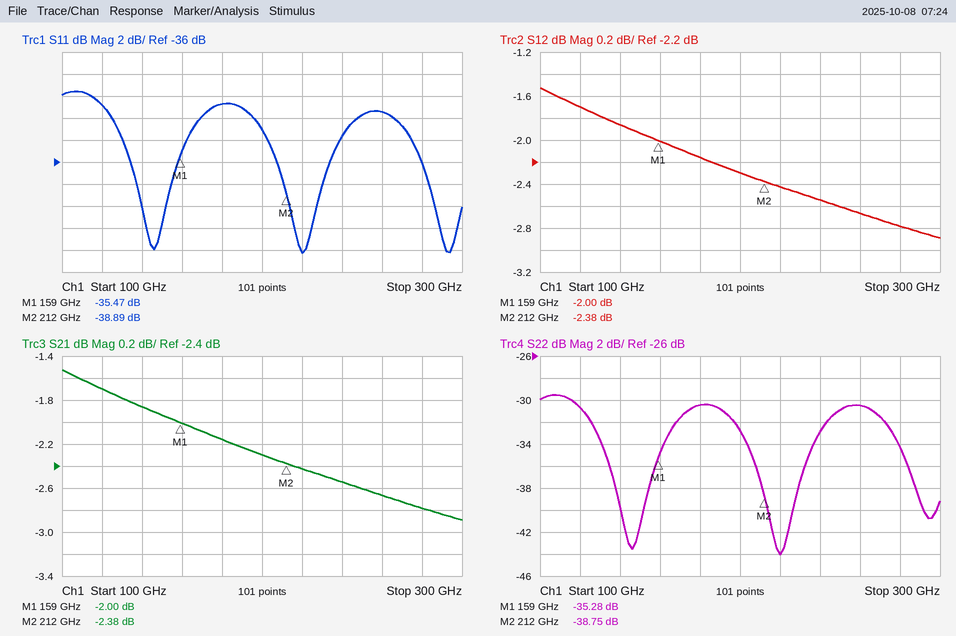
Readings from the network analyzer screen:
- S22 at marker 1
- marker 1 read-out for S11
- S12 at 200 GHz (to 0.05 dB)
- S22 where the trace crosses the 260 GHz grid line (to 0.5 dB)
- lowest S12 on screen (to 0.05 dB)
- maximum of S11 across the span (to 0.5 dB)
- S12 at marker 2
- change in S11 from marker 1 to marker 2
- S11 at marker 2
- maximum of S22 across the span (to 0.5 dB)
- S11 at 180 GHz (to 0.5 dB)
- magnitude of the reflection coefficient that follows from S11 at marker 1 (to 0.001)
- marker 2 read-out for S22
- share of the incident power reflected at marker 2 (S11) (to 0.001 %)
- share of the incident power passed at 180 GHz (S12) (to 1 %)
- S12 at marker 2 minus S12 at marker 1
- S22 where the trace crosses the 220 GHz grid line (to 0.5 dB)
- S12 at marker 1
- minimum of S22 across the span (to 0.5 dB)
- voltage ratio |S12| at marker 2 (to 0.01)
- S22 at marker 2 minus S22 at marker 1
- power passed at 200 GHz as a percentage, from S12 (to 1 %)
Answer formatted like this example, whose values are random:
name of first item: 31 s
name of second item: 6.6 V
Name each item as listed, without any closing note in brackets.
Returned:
S22 at marker 1: -35.28 dB
marker 1 read-out for S11: -35.47 dB
S12 at 200 GHz: -2.30 dB
S22 where the trace crosses the 260 GHz grid line: -30.5 dB
lowest S12 on screen: -2.90 dB
maximum of S11 across the span: -29.5 dB
S12 at marker 2: -2.38 dB
change in S11 from marker 1 to marker 2: -3.42 dB
S11 at marker 2: -38.89 dB
maximum of S22 across the span: -29.5 dB
S11 at 180 GHz: -30.5 dB
magnitude of the reflection coefficient that follows from S11 at marker 1: 0.017
marker 2 read-out for S22: -38.75 dB
share of the incident power reflected at marker 2 (S11): 0.013 %
share of the incident power passed at 180 GHz (S12): 61 %
S12 at marker 2 minus S12 at marker 1: -0.38 dB
S22 where the trace crosses the 220 GHz grid line: -44.0 dB
S12 at marker 1: -2.00 dB
minimum of S22 across the span: -44.0 dB
voltage ratio |S12| at marker 2: 0.76
S22 at marker 2 minus S22 at marker 1: -3.47 dB
power passed at 200 GHz as a percentage, from S12: 59 %
